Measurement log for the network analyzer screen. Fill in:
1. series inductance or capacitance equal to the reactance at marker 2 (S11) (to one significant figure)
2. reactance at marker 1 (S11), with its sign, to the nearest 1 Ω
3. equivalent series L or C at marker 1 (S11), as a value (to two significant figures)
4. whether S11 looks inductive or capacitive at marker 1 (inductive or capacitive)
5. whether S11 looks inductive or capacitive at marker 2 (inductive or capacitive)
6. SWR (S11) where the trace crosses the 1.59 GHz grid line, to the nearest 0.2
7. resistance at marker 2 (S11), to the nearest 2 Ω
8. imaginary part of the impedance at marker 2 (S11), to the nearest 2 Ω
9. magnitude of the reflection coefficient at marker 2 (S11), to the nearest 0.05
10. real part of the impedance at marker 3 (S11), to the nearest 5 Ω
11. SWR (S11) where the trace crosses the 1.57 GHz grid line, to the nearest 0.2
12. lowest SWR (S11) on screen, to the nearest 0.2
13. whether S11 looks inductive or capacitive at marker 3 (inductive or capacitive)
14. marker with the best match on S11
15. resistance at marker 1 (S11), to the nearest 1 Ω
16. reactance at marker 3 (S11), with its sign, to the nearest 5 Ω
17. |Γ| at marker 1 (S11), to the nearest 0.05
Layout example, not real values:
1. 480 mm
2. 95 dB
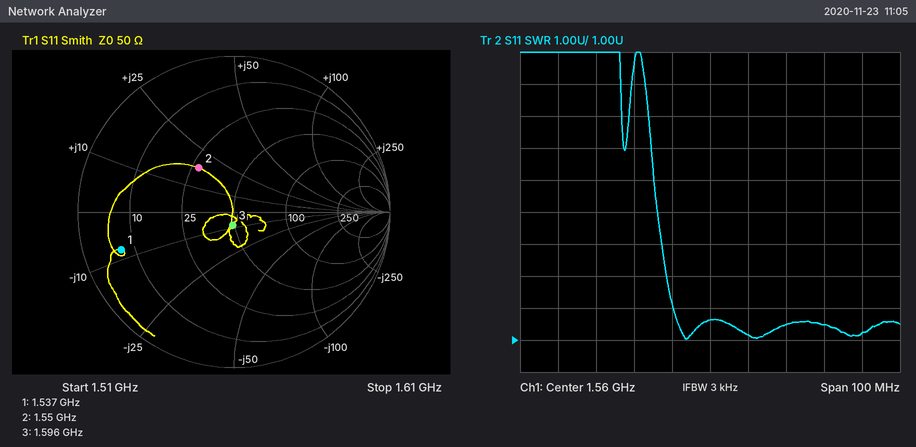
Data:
1. 2 nH
2. -8 Ω
3. 13 pF
4. capacitive
5. inductive
6. 1.4
7. 28 Ω
8. +18 Ω
9. 0.35
10. 50 Ω
11. 1.2
12. 1.0
13. capacitive
14. marker 3
15. 7 Ω
16. -10 Ω
17. 0.75
